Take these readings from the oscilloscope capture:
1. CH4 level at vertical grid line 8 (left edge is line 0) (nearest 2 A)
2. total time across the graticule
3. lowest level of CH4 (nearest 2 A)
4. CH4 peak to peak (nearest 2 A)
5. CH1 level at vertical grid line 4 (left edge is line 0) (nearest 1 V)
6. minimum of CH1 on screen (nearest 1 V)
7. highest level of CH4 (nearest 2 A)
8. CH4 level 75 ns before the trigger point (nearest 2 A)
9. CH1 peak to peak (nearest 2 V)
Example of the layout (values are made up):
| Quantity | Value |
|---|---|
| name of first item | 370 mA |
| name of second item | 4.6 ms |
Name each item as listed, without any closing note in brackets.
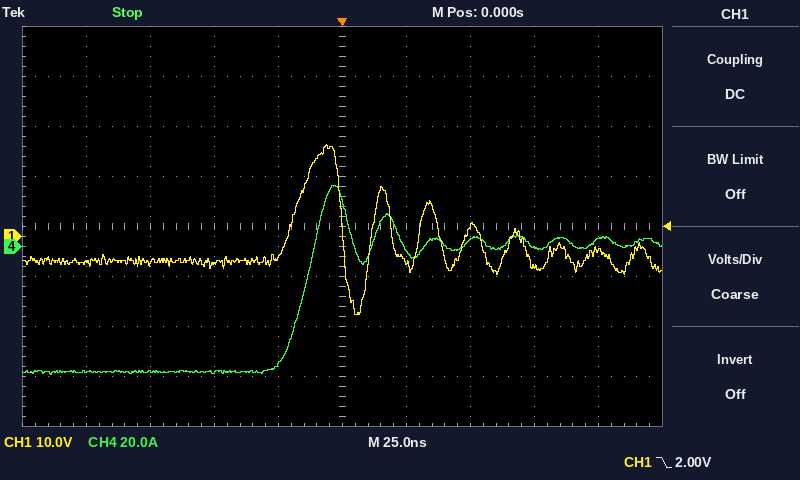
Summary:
| Quantity | Value |
|---|---|
| CH4 level at vertical grid line 8 (left edge is line 0) | 0 A |
| total time across the graticule | 250 ns |
| lowest level of CH4 | -52 A |
| CH4 peak to peak | 76 A |
| CH1 level at vertical grid line 4 (left edge is line 0) | -4 V |
| minimum of CH1 on screen | -16 V |
| highest level of CH4 | 24 A |
| CH4 level 75 ns before the trigger point | -50 A |
| CH1 peak to peak | 34 V |
